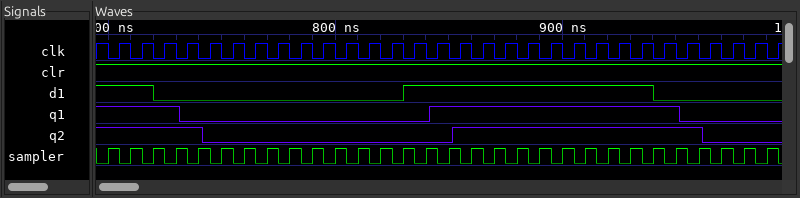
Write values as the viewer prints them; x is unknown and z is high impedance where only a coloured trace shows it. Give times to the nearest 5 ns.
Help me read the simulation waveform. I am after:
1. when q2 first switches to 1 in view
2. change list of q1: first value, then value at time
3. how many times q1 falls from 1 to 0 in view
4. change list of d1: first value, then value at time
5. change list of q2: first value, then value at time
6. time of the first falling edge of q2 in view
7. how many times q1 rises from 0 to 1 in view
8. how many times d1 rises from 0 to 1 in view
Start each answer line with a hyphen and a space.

- 850 ns
- 1, 0 at 730 ns, 1 at 840 ns, 0 at 950 ns
- 2
- 1, 0 at 720 ns, 1 at 830 ns, 0 at 940 ns
- 1, 0 at 740 ns, 1 at 850 ns, 0 at 960 ns
- 740 ns
- 1
- 1
